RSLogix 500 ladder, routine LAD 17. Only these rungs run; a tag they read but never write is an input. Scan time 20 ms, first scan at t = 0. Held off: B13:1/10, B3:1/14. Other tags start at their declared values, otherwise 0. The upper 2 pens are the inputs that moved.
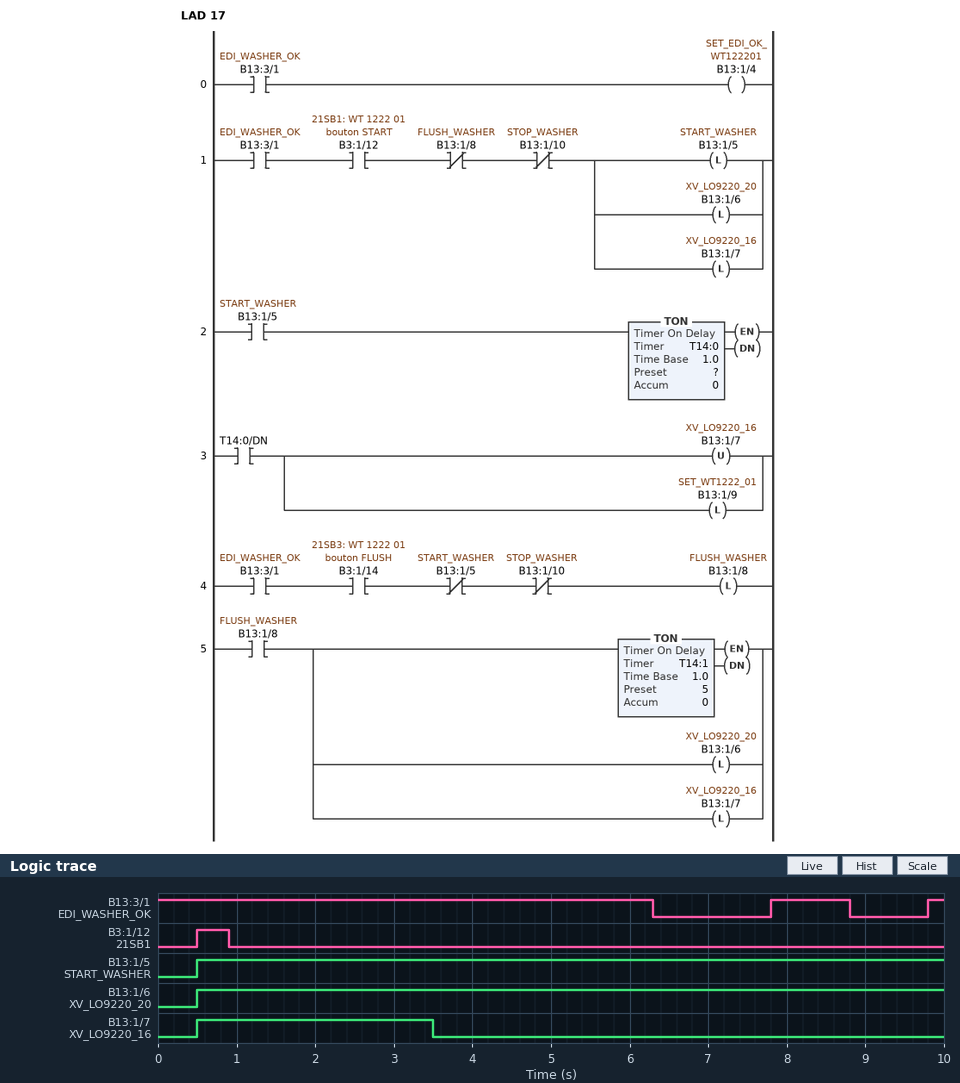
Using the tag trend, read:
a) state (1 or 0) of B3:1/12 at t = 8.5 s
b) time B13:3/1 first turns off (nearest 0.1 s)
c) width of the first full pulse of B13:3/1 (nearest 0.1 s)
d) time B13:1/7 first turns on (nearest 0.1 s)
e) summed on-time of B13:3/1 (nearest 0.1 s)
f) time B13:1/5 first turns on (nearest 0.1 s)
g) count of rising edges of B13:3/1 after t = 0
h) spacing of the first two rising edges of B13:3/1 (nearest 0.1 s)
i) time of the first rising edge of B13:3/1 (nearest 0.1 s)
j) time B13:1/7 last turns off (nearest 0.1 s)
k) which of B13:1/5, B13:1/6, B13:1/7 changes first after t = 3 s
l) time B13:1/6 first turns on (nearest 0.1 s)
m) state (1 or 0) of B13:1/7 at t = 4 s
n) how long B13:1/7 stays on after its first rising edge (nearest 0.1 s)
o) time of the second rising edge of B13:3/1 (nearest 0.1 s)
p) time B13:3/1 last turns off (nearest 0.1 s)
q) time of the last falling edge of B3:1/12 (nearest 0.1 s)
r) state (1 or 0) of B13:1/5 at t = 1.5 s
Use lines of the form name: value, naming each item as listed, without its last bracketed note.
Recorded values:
state (1 or 0) of B3:1/12 at t = 8.5 s: 0
time B13:3/1 first turns off: 6.3 s
width of the first full pulse of B13:3/1: 1.0 s
time B13:1/7 first turns on: 0.5 s
summed on-time of B13:3/1: 7.5 s
time B13:1/5 first turns on: 0.5 s
count of rising edges of B13:3/1 after t = 0: 2
spacing of the first two rising edges of B13:3/1: 2.0 s
time of the first rising edge of B13:3/1: 7.8 s
time B13:1/7 last turns off: 3.5 s
which of B13:1/5, B13:1/6, B13:1/7 changes first after t = 3 s: B13:1/7
time B13:1/6 first turns on: 0.5 s
state (1 or 0) of B13:1/7 at t = 4 s: 0
how long B13:1/7 stays on after its first rising edge: 3.0 s
time of the second rising edge of B13:3/1: 9.8 s
time B13:3/1 last turns off: 8.8 s
time of the last falling edge of B3:1/12: 0.9 s
state (1 or 0) of B13:1/5 at t = 1.5 s: 1
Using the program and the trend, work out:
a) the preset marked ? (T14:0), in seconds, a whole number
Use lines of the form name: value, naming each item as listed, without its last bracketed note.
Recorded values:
the preset marked ? (T14:0), in seconds, a whole number: 3 s
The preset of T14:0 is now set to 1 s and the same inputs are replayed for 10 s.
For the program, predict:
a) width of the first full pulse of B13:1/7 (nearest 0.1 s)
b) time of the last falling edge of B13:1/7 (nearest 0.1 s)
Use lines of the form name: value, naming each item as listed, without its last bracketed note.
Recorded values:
width of the first full pulse of B13:1/7: 1.0 s
time of the last falling edge of B13:1/7: 1.5 s
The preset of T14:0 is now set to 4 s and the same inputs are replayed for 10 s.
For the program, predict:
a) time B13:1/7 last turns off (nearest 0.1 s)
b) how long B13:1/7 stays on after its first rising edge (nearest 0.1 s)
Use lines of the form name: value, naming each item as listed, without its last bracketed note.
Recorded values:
time B13:1/7 last turns off: 4.5 s
how long B13:1/7 stays on after its first rising edge: 4.0 s
